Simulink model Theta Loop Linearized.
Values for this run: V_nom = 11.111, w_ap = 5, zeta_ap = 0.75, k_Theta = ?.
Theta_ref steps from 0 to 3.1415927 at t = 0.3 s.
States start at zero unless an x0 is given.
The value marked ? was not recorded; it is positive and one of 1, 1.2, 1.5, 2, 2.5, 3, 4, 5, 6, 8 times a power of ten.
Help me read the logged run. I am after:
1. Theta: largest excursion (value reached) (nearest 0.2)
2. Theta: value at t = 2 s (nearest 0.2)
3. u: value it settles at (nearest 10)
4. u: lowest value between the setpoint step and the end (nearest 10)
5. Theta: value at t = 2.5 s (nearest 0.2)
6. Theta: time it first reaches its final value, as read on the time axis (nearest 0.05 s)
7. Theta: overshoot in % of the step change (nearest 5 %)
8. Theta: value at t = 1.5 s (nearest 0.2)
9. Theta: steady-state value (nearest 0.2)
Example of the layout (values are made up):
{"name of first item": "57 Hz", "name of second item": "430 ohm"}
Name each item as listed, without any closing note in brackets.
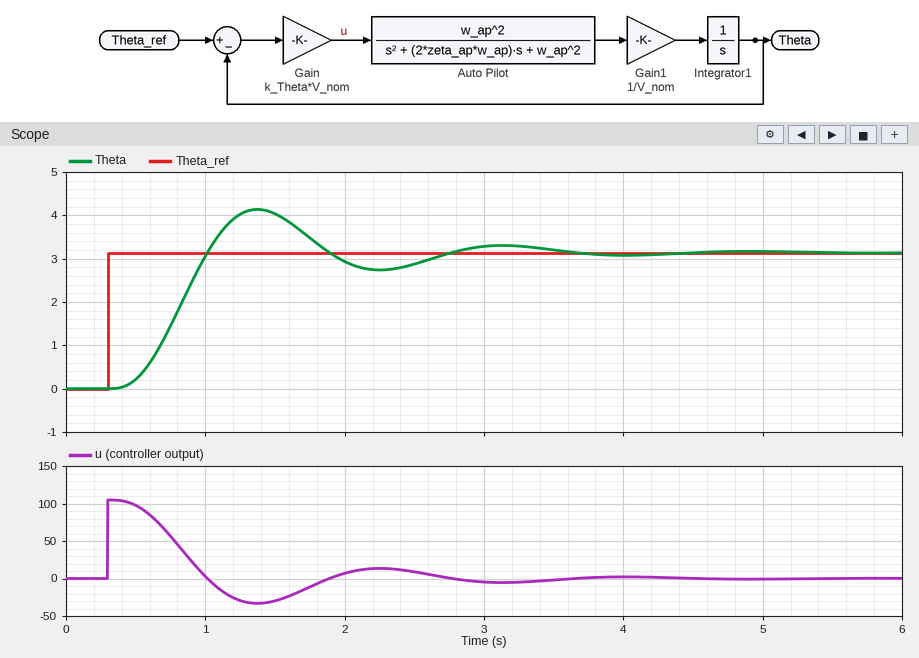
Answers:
{"Theta: largest excursion (value reached)": "4.2", "Theta: value at t = 2 s": "3.0", "u: value it settles at": "0", "u: lowest value between the setpoint step and the end": "-30", "Theta: value at t = 2.5 s": "2.8", "Theta: time it first reaches its final value, as read on the time axis": "1.00 s", "Theta: overshoot in % of the step change": "30 %", "Theta: value at t = 1.5 s": "4.0", "Theta: steady-state value": "3.2"}
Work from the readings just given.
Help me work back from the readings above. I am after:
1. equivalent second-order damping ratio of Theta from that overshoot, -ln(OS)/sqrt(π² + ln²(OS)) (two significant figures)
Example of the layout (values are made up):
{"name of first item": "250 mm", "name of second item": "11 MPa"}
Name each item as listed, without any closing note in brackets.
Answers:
{"equivalent second-order damping ratio of Theta from that overshoot, -ln(OS)/sqrt(π² + ln²(OS))": "0.36"}
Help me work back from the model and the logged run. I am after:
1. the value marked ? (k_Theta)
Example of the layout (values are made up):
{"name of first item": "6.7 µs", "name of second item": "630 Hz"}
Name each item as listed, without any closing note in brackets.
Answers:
{"the value marked ?": "3"}
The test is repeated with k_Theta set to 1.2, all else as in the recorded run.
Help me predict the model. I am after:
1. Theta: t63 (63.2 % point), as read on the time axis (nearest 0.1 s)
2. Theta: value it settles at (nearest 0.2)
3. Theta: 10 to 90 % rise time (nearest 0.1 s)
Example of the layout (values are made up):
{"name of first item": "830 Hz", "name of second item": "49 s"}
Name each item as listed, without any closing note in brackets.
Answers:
{"Theta: t63 (63.2 % point), as read on the time axis": "1.2 s", "Theta: value it settles at": "3.2", "Theta: 10 to 90 % rise time": "1.1 s"}
